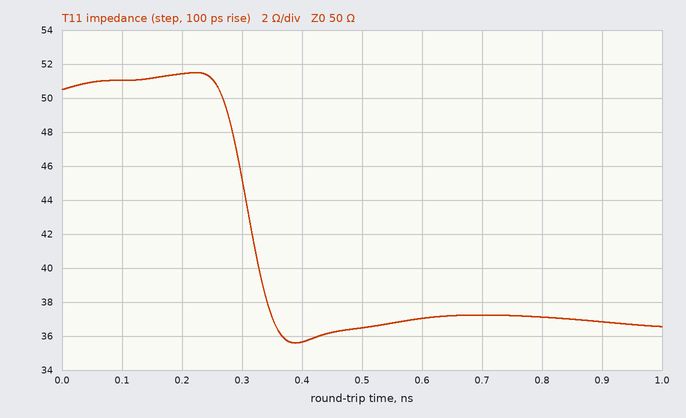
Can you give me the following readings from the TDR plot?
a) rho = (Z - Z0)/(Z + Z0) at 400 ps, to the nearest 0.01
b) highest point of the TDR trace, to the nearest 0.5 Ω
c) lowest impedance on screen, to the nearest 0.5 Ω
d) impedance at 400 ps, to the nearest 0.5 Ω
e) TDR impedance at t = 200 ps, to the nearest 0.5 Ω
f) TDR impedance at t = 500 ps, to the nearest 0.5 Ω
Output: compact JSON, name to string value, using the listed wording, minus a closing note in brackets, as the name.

{"rho = (Z - Z0)/(Z + Z0) at 400 ps, to the nearest 0.01": "-0.17", "highest point of the TDR trace, to the nearest 0.5 Ω": "51.5 Ω", "lowest impedance on screen, to the nearest 0.5 Ω": "35.5 Ω", "impedance at 400 ps, to the nearest 0.5 Ω": "35.5 Ω", "TDR impedance at t = 200 ps, to the nearest 0.5 Ω": "51.5 Ω", "TDR impedance at t = 500 ps, to the nearest 0.5 Ω": "36.5 Ω"}
